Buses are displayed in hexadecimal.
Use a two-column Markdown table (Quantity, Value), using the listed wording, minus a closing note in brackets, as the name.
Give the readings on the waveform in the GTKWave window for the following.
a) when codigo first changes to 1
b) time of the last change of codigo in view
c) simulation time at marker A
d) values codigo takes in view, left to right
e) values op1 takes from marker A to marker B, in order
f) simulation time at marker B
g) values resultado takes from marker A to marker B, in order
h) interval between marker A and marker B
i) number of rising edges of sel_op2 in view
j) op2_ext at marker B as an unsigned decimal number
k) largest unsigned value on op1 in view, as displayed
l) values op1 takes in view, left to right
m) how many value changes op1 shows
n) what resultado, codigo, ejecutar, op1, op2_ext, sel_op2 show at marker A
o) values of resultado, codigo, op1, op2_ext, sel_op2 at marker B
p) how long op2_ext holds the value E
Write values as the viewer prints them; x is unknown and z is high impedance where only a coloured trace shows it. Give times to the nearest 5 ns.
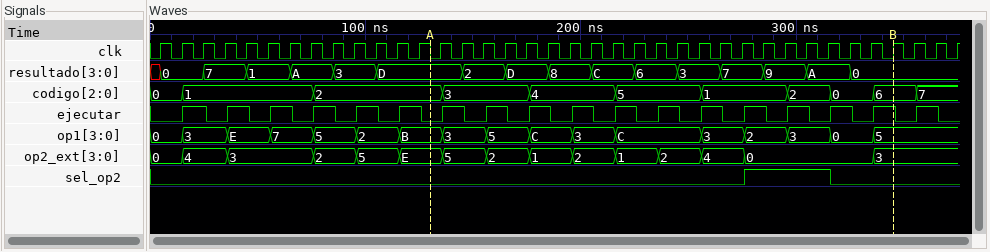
| Quantity | Value |
|---|---|
| when codigo first changes to 1 | 15 ns |
| time of the last change of codigo in view | 355 ns |
| simulation time at marker A | 130 ns |
| values codigo takes in view, left to right | 0, 1, 2, 3, 4, 5, 1, 2, 0, 6, 7 |
| values op1 takes from marker A to marker B, in order | B, 3, 5, C, 3, C, 3, 2, 3, 0, 5 |
| simulation time at marker B | 345 ns |
| values resultado takes from marker A to marker B, in order | D, 2, D, 8, C, 6, 3, 7, 9, A, 0 |
| interval between marker A and marker B | 215 ns |
| number of rising edges of sel_op2 in view | 1 |
| op2_ext at marker B as an unsigned decimal number | 3 |
| largest unsigned value on op1 in view, as displayed | E |
| values op1 takes in view, left to right | 0, 3, E, 7, 5, 2, B, 3, 5, C, 3, C, 3, 2, 3, 0, 5 |
| how many value changes op1 shows | 16 |
| what resultado, codigo, ejecutar, op1, op2_ext, sel_op2 show at marker A | resultado=D, codigo=2, ejecutar=0, op1=B, op2_ext=E, sel_op2=0 |
| values of resultado, codigo, op1, op2_ext, sel_op2 at marker B | resultado=0, codigo=6, op1=5, op2_ext=3, sel_op2=0 |
| how long op2_ext holds the value E | 20 ns |
